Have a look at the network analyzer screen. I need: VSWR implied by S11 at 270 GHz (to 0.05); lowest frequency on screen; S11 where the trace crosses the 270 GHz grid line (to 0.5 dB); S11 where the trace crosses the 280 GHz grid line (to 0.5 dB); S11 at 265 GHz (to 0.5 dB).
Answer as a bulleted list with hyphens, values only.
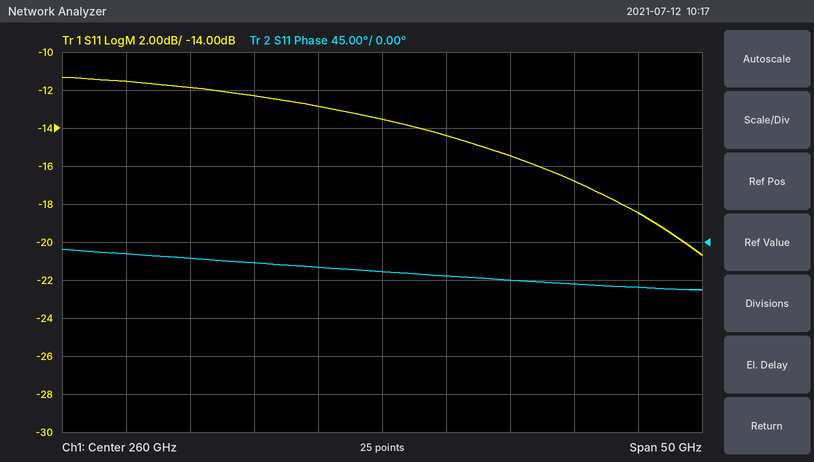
- 1.40
- 235 GHz
- -15.5 dB
- -18.5 dB
- -14.5 dB
